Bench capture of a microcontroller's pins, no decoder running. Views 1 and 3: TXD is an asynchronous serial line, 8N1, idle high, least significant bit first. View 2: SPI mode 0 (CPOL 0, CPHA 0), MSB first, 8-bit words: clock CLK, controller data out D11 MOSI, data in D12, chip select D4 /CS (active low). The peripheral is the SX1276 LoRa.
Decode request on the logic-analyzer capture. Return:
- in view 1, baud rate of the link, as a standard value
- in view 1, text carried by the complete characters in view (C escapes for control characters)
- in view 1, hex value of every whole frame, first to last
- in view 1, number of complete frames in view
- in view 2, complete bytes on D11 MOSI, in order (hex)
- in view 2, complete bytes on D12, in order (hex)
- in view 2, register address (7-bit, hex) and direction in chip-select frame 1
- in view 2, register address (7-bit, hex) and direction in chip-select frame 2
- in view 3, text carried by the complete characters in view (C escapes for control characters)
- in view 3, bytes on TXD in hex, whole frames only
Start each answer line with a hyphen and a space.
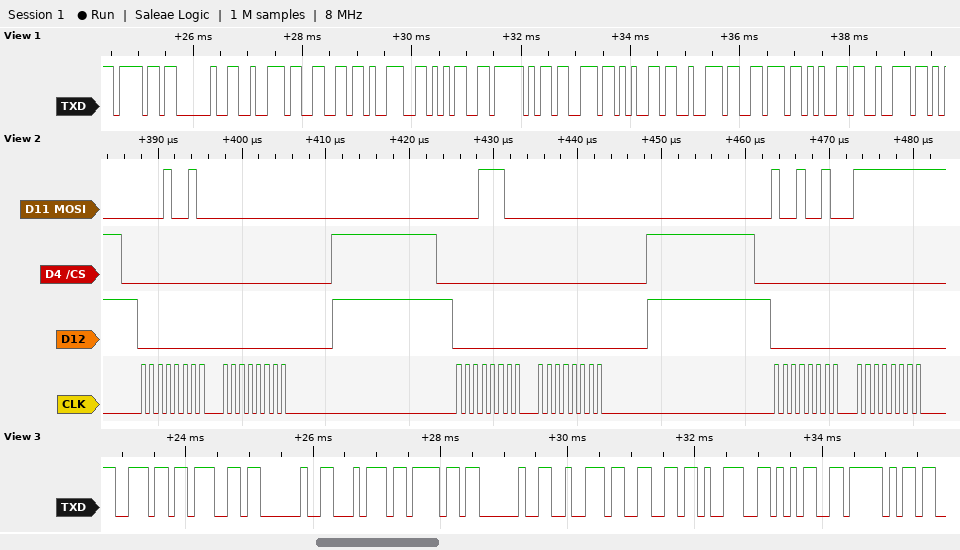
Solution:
- 9600 baud
- "o rf95_server"
- 0x6F 0x20 0x72 0x66 0x39 0x35 0x5F 0x73 0x65 0x72 0x76 0x65 0x72
- 13
- 12 00 1C 00 92 FF
- 00 00 00 00 00 00
- 0x12 read
- 0x1C read
- "ng to rf95_"
- 6E 67 20 74 6F 20 72 66 39 35 5F
